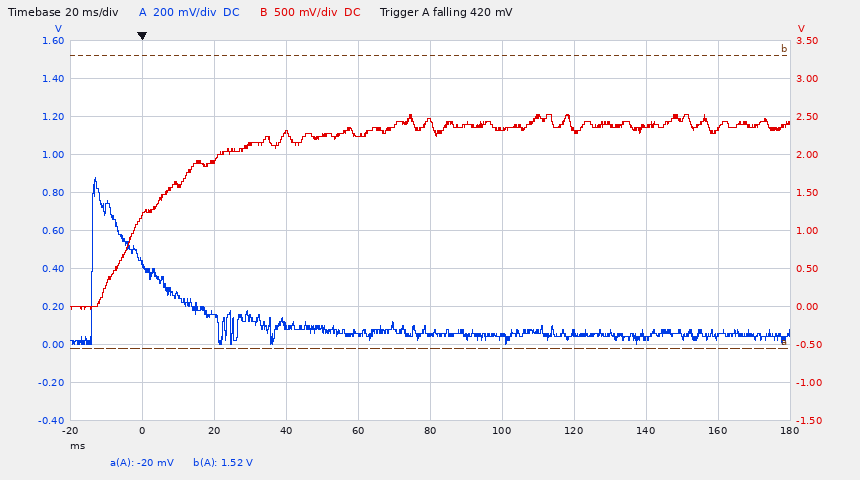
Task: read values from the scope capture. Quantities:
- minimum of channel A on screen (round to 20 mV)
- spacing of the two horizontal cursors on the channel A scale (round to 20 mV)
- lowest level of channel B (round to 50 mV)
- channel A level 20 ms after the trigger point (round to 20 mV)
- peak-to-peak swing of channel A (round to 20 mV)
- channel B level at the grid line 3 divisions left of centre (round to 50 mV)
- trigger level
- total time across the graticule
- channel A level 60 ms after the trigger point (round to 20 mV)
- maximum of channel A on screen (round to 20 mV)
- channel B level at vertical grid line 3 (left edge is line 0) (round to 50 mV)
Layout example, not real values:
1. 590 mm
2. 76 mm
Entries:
1. 0 mV
2. 1.54 V
3. -50 mV
4. 160 mV
5. 880 mV
6. 1.90 V
7. 420 mV
8. 200 ms
9. 60 mV
10. 880 mV
11. 2.30 V
